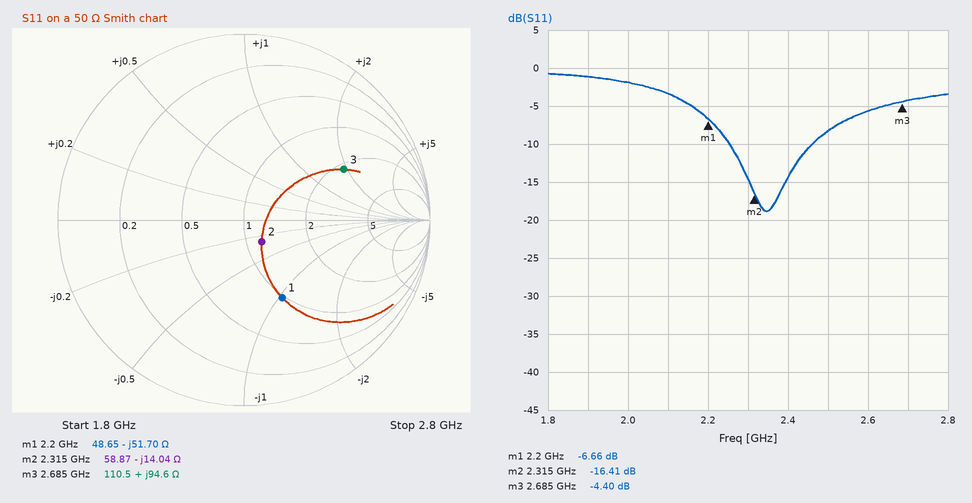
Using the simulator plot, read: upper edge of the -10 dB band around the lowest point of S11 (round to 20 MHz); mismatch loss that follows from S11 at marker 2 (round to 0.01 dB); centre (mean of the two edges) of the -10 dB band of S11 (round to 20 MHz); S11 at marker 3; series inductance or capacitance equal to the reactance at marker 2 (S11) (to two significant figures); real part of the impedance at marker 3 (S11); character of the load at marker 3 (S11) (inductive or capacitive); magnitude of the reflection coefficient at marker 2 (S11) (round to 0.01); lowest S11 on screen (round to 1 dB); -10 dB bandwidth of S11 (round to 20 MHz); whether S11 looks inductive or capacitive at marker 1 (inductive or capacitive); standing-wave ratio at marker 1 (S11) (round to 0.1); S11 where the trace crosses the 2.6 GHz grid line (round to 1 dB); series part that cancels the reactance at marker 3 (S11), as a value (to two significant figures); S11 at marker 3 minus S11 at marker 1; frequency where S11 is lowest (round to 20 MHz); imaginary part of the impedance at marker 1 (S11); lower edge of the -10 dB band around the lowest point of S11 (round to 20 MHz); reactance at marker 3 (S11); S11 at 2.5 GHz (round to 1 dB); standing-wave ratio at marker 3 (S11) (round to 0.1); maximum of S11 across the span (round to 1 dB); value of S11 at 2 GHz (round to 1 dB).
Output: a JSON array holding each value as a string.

["2.46 GHz", "0.10 dB", "2.36 GHz", "-4.40 dB", "4.9 pF", "110.5 Ω", "inductive", "0.15", "-19 dB", "200 MHz", "capacitive", "2.7", "-6 dB", "630 fF", "2.26 dB", "2.34 GHz", "-51.70 Ω", "2.26 GHz", "+94.6 Ω", "-8 dB", "4.0", "-1 dB", "-2 dB"]
